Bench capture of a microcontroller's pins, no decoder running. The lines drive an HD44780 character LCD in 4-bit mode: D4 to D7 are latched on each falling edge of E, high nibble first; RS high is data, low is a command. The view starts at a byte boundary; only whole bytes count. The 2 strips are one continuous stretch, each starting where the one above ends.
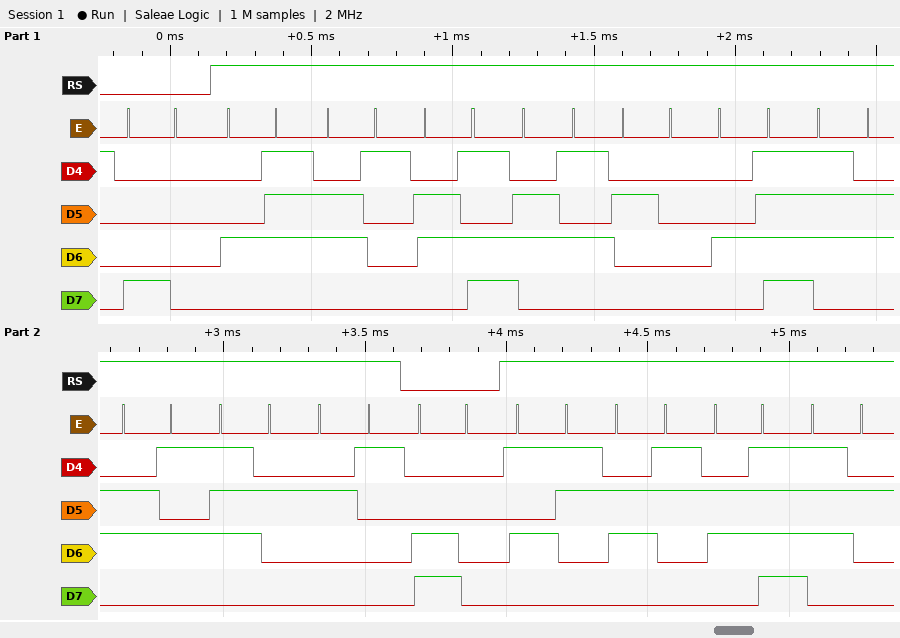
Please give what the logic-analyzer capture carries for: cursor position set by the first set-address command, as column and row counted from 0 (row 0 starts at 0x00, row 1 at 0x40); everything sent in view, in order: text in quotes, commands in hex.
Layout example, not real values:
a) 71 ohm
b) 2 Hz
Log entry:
a) column 0, row 0
b) 0x80 "Game Over!" 0xC0 "Scor"
